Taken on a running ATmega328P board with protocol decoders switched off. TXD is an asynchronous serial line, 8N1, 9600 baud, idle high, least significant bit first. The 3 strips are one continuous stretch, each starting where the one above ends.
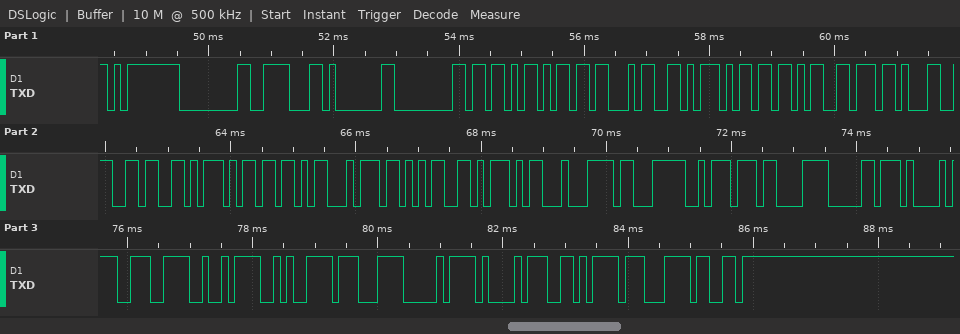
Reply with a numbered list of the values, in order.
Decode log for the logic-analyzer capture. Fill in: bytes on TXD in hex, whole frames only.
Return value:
1. 0xFD 0x00 0x1E 0x01 0x00 0x5B 0x6D 0x34 0x5D 0x5B 0x76 0x31 0x36 0x5D 0x5B 0x74 0x35 0x5D 0xC4 0xE3 0xBA 0xC3 0xB0 0xA1 0xCE 0xD2 0xCA 0xC7 0xD0 0xA1 0xD6 0xC7 0xB3
